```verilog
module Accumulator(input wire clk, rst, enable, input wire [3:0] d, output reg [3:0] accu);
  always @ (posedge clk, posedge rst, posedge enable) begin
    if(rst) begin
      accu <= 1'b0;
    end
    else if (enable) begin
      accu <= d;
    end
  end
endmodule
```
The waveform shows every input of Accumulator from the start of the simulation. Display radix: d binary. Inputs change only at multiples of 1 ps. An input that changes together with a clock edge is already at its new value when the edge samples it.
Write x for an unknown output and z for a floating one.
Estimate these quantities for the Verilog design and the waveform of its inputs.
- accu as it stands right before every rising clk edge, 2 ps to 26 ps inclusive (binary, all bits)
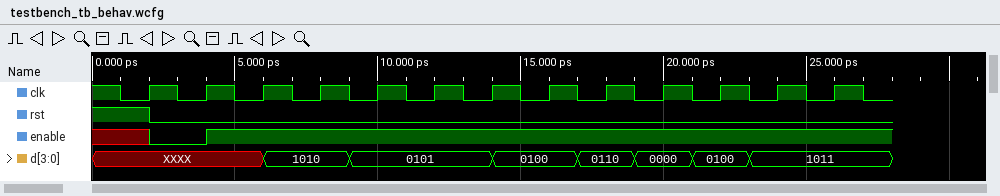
0000, 0000, x, 1010, 1010, 0101, 0101, 0100, 0100, 0110, 0000, 0100, 1011
